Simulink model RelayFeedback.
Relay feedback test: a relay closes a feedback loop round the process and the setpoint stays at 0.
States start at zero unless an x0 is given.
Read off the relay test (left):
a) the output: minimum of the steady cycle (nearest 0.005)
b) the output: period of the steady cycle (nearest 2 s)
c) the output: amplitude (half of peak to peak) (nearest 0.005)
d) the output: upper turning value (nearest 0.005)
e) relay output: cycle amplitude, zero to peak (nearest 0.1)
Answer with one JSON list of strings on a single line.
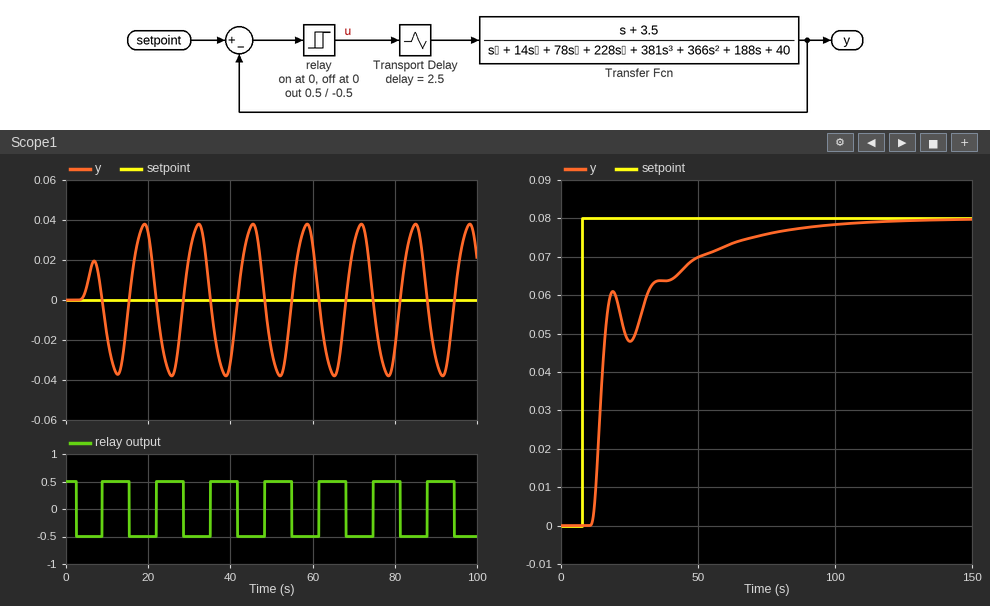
["-0.040", "14 s", "0.040", "0.040", "0.5"]
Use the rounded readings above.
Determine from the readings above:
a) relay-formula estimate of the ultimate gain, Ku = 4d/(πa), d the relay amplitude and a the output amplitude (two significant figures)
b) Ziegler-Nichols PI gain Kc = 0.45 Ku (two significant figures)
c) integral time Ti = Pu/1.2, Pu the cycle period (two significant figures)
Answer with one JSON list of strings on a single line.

["16", "7.2", "12 s"]
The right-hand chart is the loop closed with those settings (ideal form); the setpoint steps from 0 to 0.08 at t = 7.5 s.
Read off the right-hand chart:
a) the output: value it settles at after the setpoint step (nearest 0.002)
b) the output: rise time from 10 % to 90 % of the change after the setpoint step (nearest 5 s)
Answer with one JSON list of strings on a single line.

["0.080", "45 s"]
